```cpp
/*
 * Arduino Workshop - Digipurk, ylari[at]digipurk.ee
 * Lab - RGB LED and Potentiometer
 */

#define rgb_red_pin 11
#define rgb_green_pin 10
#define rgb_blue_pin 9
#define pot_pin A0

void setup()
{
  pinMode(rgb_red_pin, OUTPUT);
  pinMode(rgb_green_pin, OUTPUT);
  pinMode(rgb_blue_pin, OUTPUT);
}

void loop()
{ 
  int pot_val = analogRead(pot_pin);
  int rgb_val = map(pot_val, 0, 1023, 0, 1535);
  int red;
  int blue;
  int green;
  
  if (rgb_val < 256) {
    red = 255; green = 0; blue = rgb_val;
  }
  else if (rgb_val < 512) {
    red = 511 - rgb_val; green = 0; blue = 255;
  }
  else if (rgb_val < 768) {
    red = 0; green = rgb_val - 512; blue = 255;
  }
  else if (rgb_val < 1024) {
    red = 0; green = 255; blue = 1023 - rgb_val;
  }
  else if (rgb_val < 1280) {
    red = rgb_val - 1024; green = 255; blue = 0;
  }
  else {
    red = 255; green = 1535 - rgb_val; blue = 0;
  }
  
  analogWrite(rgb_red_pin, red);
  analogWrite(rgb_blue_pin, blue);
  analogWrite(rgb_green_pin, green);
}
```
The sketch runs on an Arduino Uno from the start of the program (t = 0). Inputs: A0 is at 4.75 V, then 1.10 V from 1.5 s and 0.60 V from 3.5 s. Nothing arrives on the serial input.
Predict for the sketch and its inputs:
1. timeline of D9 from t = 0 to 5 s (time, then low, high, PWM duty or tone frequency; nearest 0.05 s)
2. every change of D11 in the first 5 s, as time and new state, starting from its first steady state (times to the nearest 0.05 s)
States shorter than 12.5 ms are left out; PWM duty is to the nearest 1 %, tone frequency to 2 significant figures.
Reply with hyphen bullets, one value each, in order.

- 0 s low; 1.5 s high; 3.5 s PWM 72 %
- 0 s high; 1.5 s PWM 68 %; 3.5 s high
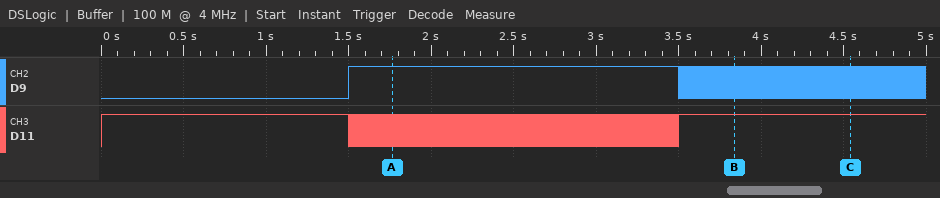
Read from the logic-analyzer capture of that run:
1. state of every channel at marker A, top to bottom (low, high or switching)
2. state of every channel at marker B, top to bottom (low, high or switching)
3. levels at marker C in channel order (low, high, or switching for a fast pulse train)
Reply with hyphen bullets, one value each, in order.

- D9 high, D11 switching
- D9 switching, D11 high
- D9 switching, D11 high
